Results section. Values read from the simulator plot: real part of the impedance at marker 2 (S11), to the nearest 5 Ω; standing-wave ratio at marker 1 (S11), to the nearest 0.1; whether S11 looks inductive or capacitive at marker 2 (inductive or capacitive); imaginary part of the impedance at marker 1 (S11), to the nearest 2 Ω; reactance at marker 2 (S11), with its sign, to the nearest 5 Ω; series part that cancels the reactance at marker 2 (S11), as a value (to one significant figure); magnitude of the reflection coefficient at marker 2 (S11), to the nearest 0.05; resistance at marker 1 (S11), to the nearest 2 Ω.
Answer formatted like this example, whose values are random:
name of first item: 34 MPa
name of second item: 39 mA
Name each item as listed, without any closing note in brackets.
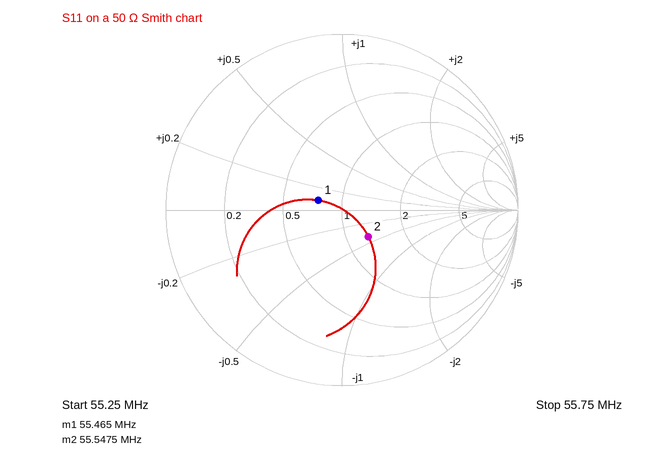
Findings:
real part of the impedance at marker 2 (S11), to the nearest 5 Ω: 65 Ω
standing-wave ratio at marker 1 (S11), to the nearest 0.1: 1.3
whether S11 looks inductive or capacitive at marker 2: capacitive
imaginary part of the impedance at marker 1 (S11), to the nearest 2 Ω: +4 Ω
reactance at marker 2 (S11), with its sign, to the nearest 5 Ω: -20 Ω
series part that cancels the reactance at marker 2 (S11), as a value: 60 nH
magnitude of the reflection coefficient at marker 2 (S11), to the nearest 0.05: 0.20
resistance at marker 1 (S11), to the nearest 2 Ω: 38 Ω
